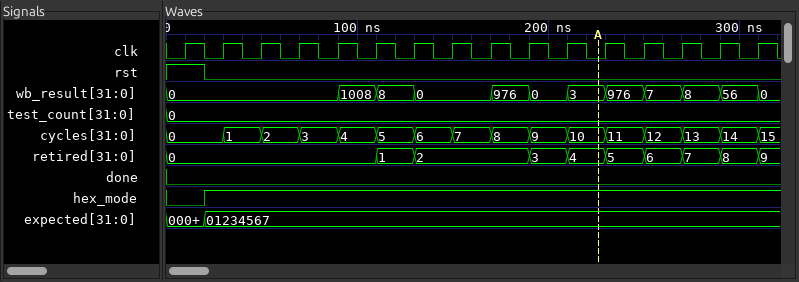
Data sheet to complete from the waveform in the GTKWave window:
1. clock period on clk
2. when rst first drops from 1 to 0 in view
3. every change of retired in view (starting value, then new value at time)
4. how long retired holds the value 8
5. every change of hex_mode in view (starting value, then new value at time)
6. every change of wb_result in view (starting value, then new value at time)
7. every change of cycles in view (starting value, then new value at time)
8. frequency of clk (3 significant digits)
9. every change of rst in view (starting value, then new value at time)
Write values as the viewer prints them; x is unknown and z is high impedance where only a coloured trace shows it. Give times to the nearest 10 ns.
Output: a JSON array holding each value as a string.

["20 ns", "20 ns", "0, 1 at 110 ns, 2 at 130 ns, 3 at 190 ns, 4 at 210 ns, 5 at 230 ns, 6 at 250 ns, 7 at 270 ns, 8 at 290 ns, 9 at 310 ns", "20 ns", "0, 1 at 20 ns", "0, 1008 at 90 ns, 8 at 110 ns, 0 at 130 ns, 976 at 170 ns, 0 at 190 ns, 3 at 210 ns, 976 at 230 ns, 7 at 250 ns, 8 at 270 ns, 56 at 290 ns, 0 at 310 ns", "0, 1 at 30 ns, 2 at 50 ns, 3 at 70 ns, 4 at 90 ns, 5 at 110 ns, 6 at 130 ns, 7 at 150 ns, 8 at 170 ns, 9 at 190 ns, 10 at 210 ns, 11 at 230 ns, 12 at 250 ns, 13 at 270 ns, 14 at 290 ns, 15 at 310 ns", "50.0 MHz", "1, 0 at 20 ns"]
